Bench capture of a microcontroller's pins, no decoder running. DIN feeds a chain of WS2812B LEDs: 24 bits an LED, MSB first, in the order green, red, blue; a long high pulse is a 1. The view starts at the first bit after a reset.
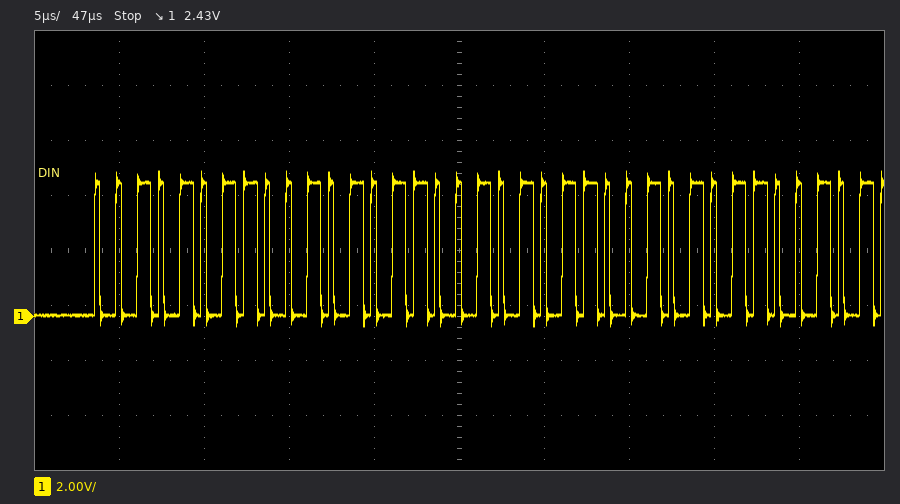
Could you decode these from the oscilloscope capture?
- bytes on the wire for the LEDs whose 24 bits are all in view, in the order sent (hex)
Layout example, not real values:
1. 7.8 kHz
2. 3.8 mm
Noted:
1. 2B 2B 2B
